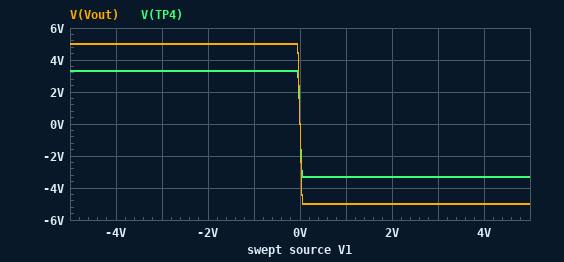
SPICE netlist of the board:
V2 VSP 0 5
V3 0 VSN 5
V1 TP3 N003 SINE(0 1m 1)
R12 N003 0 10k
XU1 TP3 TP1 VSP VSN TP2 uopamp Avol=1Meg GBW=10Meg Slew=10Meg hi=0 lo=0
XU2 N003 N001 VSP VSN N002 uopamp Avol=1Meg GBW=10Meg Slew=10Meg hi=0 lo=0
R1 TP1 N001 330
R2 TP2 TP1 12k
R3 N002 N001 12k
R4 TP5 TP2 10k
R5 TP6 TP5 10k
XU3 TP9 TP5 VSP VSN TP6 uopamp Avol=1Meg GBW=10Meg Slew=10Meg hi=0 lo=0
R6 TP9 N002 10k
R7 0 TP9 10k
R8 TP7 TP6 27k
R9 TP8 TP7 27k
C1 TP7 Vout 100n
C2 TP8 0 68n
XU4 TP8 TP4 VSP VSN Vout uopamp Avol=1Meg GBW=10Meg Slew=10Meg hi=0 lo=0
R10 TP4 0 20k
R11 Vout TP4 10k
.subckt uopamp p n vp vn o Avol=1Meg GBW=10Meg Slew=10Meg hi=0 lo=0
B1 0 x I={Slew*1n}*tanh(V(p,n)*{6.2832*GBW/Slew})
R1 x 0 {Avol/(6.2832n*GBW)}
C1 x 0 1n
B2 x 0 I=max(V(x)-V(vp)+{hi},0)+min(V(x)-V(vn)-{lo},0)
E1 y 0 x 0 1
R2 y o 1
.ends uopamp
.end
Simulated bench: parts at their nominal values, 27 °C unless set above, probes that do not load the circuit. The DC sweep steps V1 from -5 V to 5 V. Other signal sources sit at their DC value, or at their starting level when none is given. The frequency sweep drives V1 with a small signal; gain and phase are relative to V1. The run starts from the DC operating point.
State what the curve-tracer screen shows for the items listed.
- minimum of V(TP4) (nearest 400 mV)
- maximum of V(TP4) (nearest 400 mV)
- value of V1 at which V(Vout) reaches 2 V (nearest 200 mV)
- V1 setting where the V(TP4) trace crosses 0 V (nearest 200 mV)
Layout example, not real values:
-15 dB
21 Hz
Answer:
-3.2 V
3.2 V
0 V
0 V
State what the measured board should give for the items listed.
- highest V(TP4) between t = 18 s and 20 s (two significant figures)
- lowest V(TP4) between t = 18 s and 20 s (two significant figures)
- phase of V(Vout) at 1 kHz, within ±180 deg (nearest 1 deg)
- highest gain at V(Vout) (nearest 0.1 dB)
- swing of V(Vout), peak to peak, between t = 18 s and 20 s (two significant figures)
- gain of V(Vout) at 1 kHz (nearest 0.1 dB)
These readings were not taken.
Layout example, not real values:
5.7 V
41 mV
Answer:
74 mV
-74 mV
4 deg
41.9 dB
220 mV
-4.9 dB
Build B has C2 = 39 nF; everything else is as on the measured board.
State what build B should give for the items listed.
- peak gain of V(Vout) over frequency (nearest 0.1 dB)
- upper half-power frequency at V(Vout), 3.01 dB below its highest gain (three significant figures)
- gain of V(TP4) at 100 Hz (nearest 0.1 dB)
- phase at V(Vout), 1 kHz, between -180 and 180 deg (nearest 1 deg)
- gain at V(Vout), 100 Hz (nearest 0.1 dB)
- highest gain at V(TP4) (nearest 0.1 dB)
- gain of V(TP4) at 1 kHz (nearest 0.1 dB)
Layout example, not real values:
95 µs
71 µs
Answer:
48.1 dB
109 Hz
43.5 dB
2 deg
47.1 dB
44.5 dB
-3.6 dB
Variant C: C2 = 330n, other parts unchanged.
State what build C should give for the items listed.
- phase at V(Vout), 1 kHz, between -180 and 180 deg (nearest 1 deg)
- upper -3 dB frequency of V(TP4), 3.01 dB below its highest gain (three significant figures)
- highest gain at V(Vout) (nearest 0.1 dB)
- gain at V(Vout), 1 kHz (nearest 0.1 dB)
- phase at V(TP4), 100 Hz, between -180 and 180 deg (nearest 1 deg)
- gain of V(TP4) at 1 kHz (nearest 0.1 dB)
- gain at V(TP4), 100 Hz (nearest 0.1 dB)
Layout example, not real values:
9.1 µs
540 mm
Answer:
6 deg
10.6 Hz
40.9 dB
-18.7 dB
51 deg
-22.2 dB
14.8 dB
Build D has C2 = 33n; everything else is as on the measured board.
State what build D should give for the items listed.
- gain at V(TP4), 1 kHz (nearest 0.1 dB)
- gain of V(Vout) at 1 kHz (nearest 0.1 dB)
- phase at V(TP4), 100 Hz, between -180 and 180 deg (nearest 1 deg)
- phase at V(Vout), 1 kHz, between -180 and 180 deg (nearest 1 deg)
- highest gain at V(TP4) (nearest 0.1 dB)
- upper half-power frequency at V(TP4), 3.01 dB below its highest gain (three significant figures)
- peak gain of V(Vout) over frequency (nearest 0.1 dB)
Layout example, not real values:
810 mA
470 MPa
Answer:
-2.1 dB
1.4 dB
100 deg
1 deg
48.5 dB
114 Hz
52.1 dB
